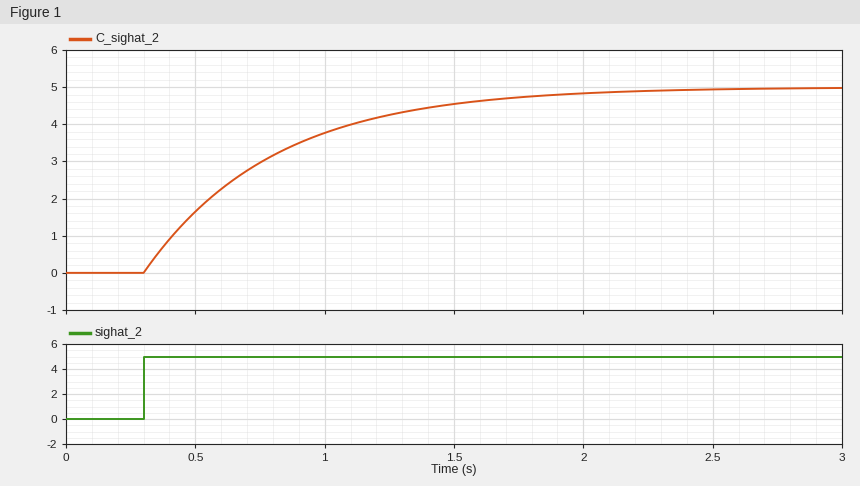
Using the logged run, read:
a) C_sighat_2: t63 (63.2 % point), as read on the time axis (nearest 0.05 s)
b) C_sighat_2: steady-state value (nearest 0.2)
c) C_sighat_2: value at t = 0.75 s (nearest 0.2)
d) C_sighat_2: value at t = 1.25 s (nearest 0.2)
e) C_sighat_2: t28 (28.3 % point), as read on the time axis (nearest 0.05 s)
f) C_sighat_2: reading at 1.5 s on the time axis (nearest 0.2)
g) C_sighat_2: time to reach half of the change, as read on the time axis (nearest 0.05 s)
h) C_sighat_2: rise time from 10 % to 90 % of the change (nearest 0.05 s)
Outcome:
0.80 s
5.0
3.0
4.2
0.45 s
4.6
0.65 s
1.10 s
